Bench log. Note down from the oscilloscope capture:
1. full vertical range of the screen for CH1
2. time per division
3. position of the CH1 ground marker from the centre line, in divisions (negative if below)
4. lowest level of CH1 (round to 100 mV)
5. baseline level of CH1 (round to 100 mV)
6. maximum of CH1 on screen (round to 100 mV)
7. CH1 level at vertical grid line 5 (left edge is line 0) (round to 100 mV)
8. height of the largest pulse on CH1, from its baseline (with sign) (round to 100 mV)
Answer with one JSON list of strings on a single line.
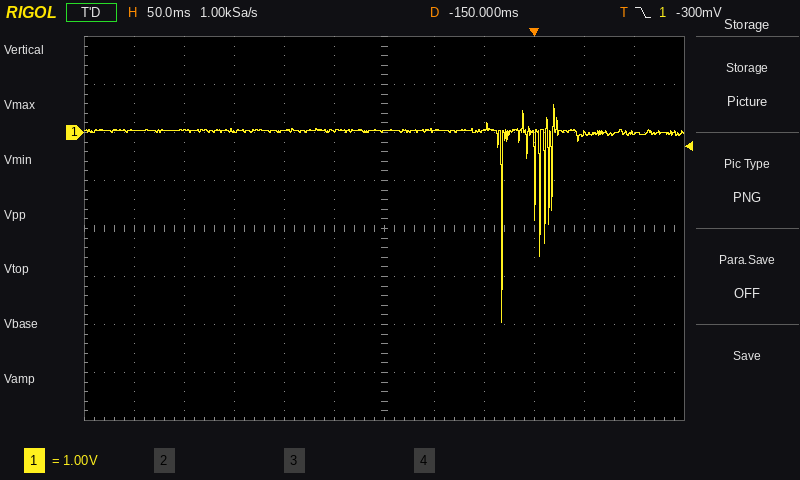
["8 V", "50 ms", "+2.0 div", "-4.0 V", "0.0 V", "600 mV", "0.0 V", "-4.0 V"]
